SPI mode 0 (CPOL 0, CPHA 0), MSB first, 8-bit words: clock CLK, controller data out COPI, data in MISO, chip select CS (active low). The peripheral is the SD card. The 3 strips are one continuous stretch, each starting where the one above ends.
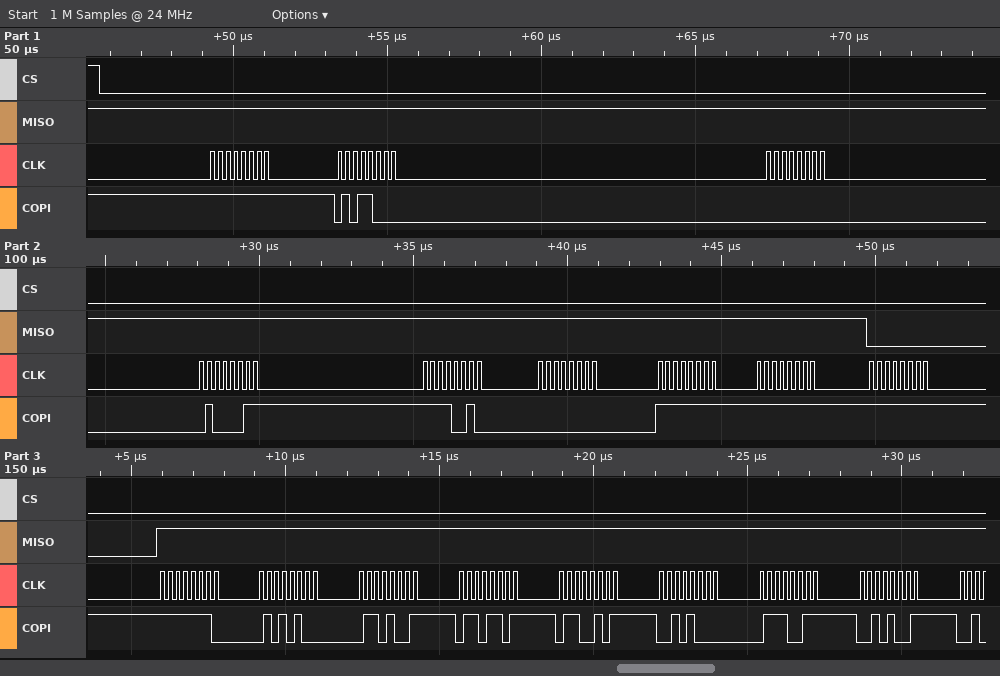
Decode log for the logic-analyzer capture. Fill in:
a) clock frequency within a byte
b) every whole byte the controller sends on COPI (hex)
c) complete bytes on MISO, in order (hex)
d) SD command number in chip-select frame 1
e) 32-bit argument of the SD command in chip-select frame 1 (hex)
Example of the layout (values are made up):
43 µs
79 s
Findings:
4 MHz
0xFF 0x58 0x00 0x43 0xF2 0x00 0xFF 0xFF 0xFF 0xFE 0x54 0x69 0x6D 0x65 0x28 0x73 0x29
0xFF 0xFF 0xFF 0xFF 0xFF 0xFF 0xFF 0xFF 0x00 0xFF 0xFF 0xFF 0xFF 0xFF 0xFF 0xFF 0xFF
CMD24
0x0043F200
